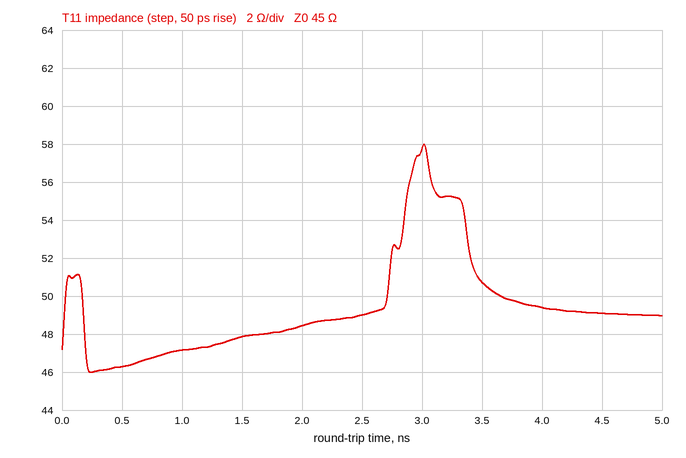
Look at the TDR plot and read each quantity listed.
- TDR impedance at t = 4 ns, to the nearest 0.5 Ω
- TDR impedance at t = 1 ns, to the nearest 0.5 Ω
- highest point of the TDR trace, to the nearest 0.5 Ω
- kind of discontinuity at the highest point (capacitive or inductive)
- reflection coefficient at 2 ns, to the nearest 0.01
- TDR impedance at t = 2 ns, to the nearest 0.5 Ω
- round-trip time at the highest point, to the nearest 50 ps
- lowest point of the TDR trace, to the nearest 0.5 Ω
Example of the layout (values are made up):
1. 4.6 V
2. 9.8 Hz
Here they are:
1. 49.5 Ω
2. 47.0 Ω
3. 58.0 Ω
4. inductive
5. +0.04
6. 48.5 Ω
7. 3.00 ns
8. 46.0 Ω
